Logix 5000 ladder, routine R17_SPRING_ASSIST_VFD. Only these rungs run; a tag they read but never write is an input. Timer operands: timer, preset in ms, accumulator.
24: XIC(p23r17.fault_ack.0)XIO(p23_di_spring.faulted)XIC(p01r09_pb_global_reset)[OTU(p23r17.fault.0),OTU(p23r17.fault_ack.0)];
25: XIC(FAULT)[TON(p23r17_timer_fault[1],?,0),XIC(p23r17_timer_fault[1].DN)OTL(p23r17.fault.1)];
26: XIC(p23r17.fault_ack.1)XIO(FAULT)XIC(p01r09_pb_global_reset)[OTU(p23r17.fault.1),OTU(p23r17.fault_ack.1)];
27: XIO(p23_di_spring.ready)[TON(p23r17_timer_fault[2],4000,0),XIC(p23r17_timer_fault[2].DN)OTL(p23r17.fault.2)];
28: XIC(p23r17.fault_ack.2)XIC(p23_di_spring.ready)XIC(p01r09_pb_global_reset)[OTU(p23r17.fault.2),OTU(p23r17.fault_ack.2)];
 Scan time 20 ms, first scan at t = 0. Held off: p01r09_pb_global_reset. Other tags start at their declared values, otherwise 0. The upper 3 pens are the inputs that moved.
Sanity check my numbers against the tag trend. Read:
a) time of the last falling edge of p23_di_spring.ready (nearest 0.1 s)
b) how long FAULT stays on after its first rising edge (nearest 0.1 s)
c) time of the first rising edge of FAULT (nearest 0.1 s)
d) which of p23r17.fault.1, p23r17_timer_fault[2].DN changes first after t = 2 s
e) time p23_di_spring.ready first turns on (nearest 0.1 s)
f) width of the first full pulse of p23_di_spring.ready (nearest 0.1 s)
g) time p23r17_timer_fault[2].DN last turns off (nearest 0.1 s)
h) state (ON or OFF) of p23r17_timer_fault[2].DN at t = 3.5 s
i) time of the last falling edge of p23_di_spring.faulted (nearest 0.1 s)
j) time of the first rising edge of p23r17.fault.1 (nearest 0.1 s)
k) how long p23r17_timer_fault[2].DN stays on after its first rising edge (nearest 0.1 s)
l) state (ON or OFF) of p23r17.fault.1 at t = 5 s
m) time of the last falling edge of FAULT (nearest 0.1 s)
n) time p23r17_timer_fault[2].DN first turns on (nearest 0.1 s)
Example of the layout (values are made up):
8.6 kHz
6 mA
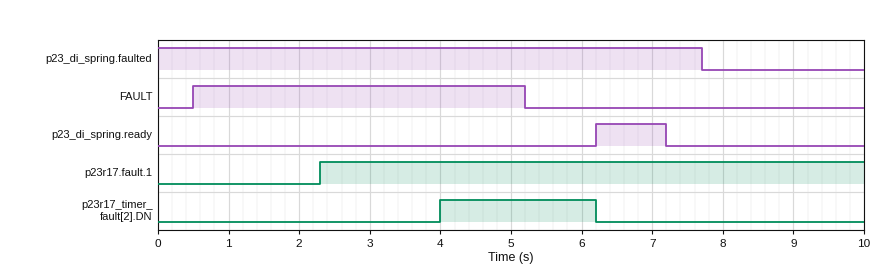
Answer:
7.2 s
4.7 s
0.5 s
p23r17.fault.1
6.2 s
1.0 s
6.2 s
OFF
7.7 s
2.3 s
2.2 s
ON
5.2 s
4.0 s
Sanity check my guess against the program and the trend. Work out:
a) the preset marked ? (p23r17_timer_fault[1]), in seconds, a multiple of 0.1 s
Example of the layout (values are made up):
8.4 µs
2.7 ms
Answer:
1.8 s
